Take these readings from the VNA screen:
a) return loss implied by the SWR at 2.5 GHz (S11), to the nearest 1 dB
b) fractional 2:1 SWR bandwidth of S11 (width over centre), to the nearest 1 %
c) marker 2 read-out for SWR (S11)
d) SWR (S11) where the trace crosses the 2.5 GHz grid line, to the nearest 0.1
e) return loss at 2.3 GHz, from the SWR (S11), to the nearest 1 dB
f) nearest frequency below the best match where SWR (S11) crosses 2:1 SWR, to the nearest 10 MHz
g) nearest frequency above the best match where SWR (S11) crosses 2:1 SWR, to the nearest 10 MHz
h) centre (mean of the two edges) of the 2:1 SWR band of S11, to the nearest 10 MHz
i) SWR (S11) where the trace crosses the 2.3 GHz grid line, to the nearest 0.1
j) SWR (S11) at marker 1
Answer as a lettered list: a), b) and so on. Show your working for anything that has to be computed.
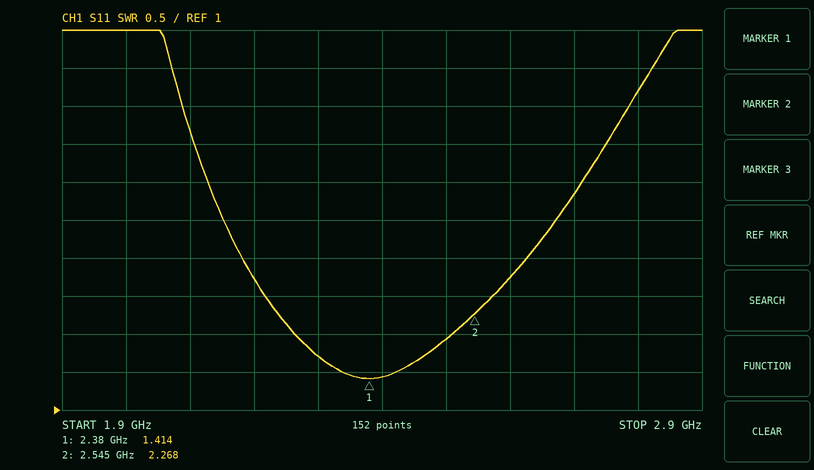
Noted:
a) −20 log10((1.9 − 1)/(1.9 + 1)) ≈ 10 dB
b) 250 MHz / 2.385 GHz ≈ 10 %
c) 2.268
d) 1.9
e) −20 log10((1.7 − 1)/(1.7 + 1)) ≈ 12 dB
f) 2.26 GHz
g) 2.51 GHz
h) 2.39 GHz
i) 1.7
j) 1.414
